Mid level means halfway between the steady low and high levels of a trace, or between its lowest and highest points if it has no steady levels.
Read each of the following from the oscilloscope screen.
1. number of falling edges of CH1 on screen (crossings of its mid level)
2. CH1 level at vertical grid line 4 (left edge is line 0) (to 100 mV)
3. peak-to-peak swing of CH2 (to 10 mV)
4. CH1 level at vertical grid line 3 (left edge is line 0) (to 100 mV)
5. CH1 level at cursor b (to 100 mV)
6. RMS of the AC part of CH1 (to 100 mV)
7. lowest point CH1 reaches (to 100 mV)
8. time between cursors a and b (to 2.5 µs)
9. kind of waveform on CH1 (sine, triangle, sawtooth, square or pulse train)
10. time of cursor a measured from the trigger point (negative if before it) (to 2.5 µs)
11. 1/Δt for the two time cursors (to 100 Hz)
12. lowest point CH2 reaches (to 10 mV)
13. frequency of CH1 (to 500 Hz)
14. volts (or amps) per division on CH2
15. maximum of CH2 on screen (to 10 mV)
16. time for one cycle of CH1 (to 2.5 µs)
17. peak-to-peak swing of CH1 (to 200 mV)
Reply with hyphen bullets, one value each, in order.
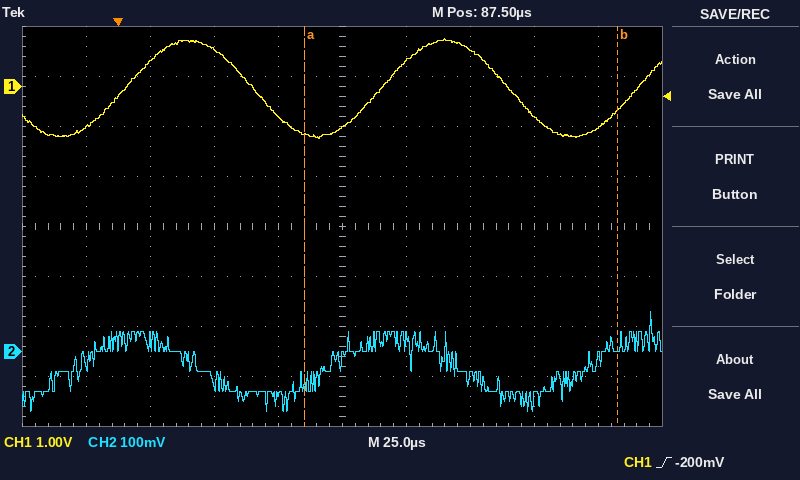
- 2
- -600 mV
- 200 mV
- 700 mV
- -500 mV
- 700 mV
- -1.0 V
- 122.5 µs
- sine
- +72.5 µs
- 8.2 kHz
- -120 mV
- 10.0 kHz
- 100 mV
- 80 mV
- 100.0 µs
- 2.0 V
